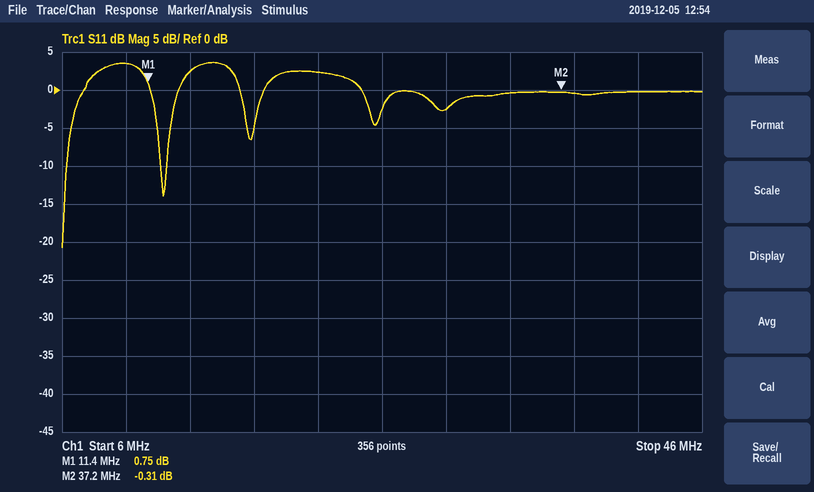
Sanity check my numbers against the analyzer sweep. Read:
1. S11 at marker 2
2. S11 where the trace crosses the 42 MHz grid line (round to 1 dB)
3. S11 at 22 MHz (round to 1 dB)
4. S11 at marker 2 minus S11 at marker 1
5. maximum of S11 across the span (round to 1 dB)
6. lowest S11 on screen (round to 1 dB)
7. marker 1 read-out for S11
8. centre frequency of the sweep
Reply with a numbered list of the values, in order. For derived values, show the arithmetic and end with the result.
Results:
1. -0.31 dB
2. 0 dB
3. 2 dB
4. -0.31 − (0.75) = -1.06 dB
5. 4 dB
6. -21 dB
7. 0.75 dB
8. 26 MHz
